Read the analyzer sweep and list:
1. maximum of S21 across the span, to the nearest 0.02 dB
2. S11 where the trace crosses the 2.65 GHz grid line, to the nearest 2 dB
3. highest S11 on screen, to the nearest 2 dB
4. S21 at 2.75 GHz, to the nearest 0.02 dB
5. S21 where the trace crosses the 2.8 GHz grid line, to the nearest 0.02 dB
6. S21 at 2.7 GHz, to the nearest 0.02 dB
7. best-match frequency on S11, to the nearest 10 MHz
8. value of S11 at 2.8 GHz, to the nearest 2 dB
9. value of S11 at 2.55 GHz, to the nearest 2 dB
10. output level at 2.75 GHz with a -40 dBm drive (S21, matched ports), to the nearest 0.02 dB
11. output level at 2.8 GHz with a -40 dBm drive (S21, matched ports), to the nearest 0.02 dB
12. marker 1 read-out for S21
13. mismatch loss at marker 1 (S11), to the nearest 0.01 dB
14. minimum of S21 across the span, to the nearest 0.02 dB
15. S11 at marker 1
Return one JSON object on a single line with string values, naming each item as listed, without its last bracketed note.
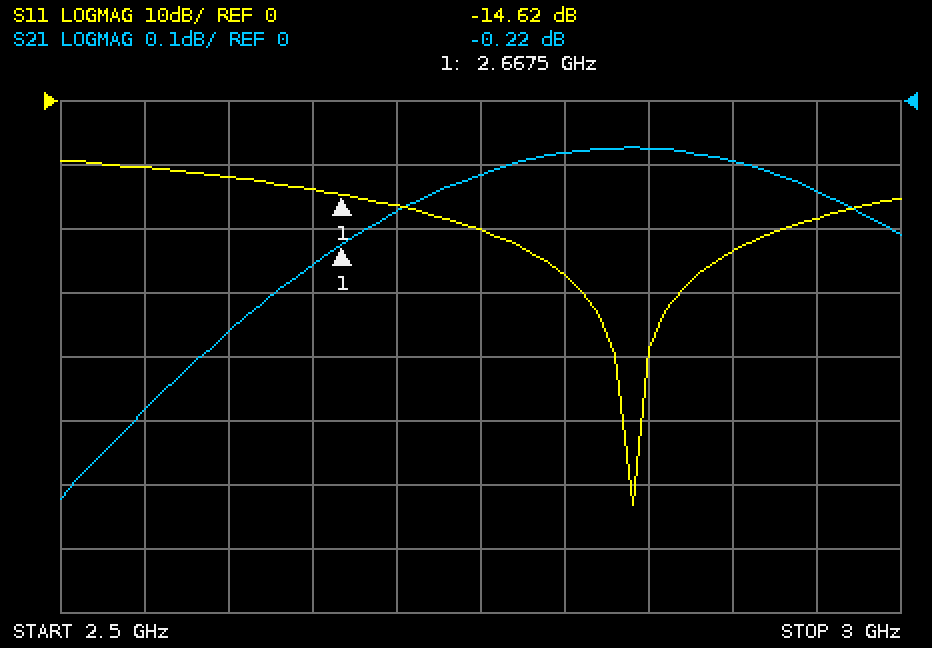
{"maximum of S21 across the span, to the nearest 0.02 dB": "-0.08 dB", "S11 where the trace crosses the 2.65 GHz grid line, to the nearest 2 dB": "-14 dB", "highest S11 on screen, to the nearest 2 dB": "-10 dB", "S21 at 2.75 GHz, to the nearest 0.02 dB": "-0.12 dB", "S21 where the trace crosses the 2.8 GHz grid line, to the nearest 0.02 dB": "-0.08 dB", "S21 at 2.7 GHz, to the nearest 0.02 dB": "-0.18 dB", "best-match frequency on S11, to the nearest 10 MHz": "2.84 GHz", "value of S11 at 2.8 GHz, to the nearest 2 dB": "-28 dB", "value of S11 at 2.55 GHz, to the nearest 2 dB": "-10 dB", "output level at 2.75 GHz with a -40 dBm drive (S21, matched ports), to the nearest 0.02 dB": "-40.12 dBm", "output level at 2.8 GHz with a -40 dBm drive (S21, matched ports), to the nearest 0.02 dB": "-40.08 dBm", "marker 1 read-out for S21": "-0.22 dB", "mismatch loss at marker 1 (S11), to the nearest 0.01 dB": "0.15 dB", "minimum of S21 across the span, to the nearest 0.02 dB": "-0.62 dB", "S11 at marker 1": "-14.62 dB"}
